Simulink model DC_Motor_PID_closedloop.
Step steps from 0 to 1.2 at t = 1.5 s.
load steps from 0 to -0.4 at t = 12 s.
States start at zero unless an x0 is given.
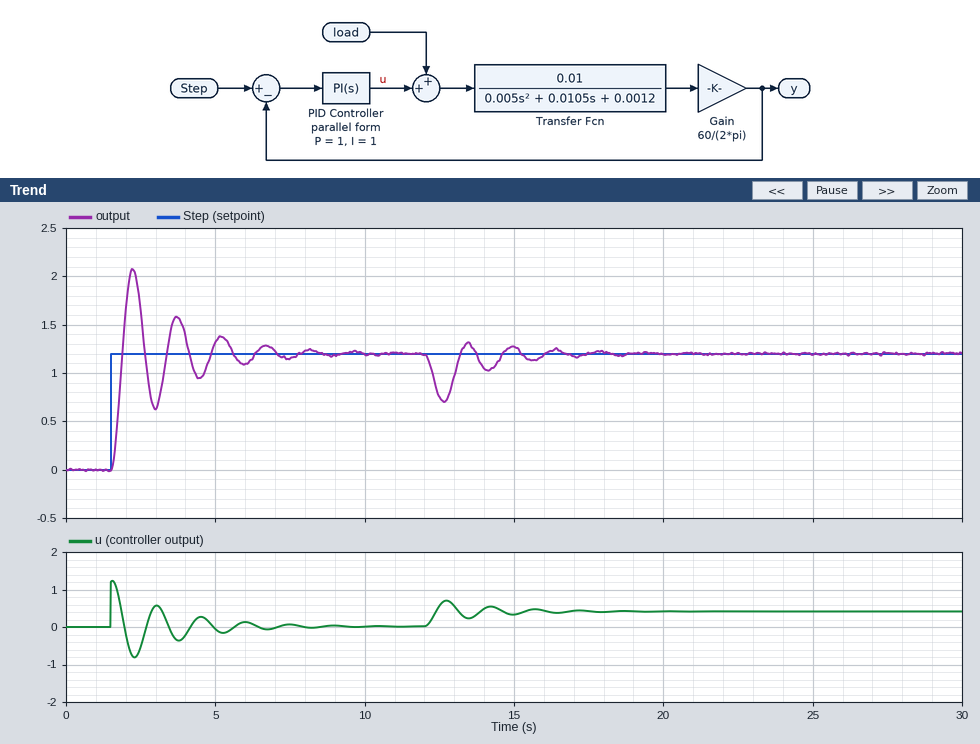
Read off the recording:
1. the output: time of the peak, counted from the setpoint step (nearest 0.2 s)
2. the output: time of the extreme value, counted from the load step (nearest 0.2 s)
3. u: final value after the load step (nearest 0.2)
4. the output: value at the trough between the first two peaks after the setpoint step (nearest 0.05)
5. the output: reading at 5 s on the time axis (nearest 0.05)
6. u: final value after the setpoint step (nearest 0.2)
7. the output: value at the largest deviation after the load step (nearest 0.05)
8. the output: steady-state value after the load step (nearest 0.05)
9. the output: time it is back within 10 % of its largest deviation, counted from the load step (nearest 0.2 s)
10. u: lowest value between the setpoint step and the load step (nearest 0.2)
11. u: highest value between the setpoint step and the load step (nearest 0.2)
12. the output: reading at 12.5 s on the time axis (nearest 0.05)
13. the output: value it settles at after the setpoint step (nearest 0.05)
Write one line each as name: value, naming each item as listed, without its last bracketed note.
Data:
the output: time of the peak, counted from the setpoint step: 0.8 s
the output: time of the extreme value, counted from the load step: 0.6 s
u: final value after the load step: 0.4
the output: value at the trough between the first two peaks after the setpoint step: 0.65
the output: reading at 5 s on the time axis: 1.30
u: final value after the setpoint step: 0.0
the output: value at the largest deviation after the load step: 0.70
the output: steady-state value after the load step: 1.20
the output: time it is back within 10 % of its largest deviation, counted from the load step: 3.8 s
u: lowest value between the setpoint step and the load step: -0.8
u: highest value between the setpoint step and the load step: 1.2
the output: reading at 12.5 s on the time axis: 0.75
the output: value it settles at after the setpoint step: 1.20
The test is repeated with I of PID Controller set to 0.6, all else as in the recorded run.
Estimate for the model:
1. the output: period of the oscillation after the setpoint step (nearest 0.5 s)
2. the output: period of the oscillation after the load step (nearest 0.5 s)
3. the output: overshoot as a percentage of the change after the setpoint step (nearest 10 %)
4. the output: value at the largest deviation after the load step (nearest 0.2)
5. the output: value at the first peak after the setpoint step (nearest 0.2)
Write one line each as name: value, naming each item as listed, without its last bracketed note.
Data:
the output: period of the oscillation after the setpoint step: 1.5 s
the output: period of the oscillation after the load step: 1.5 s
the output: overshoot as a percentage of the change after the setpoint step: 60 %
the output: value at the largest deviation after the load step: 0.6
the output: value at the first peak after the setpoint step: 2.0
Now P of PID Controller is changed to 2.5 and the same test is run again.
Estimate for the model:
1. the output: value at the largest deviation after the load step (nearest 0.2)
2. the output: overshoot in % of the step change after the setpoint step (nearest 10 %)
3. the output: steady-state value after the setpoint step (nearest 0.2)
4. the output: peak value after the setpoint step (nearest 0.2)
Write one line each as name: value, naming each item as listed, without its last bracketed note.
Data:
the output: value at the largest deviation after the load step: 1.0
the output: overshoot in % of the step change after the setpoint step: 70 %
the output: steady-state value after the setpoint step: 1.2
the output: peak value after the setpoint step: 2.0
